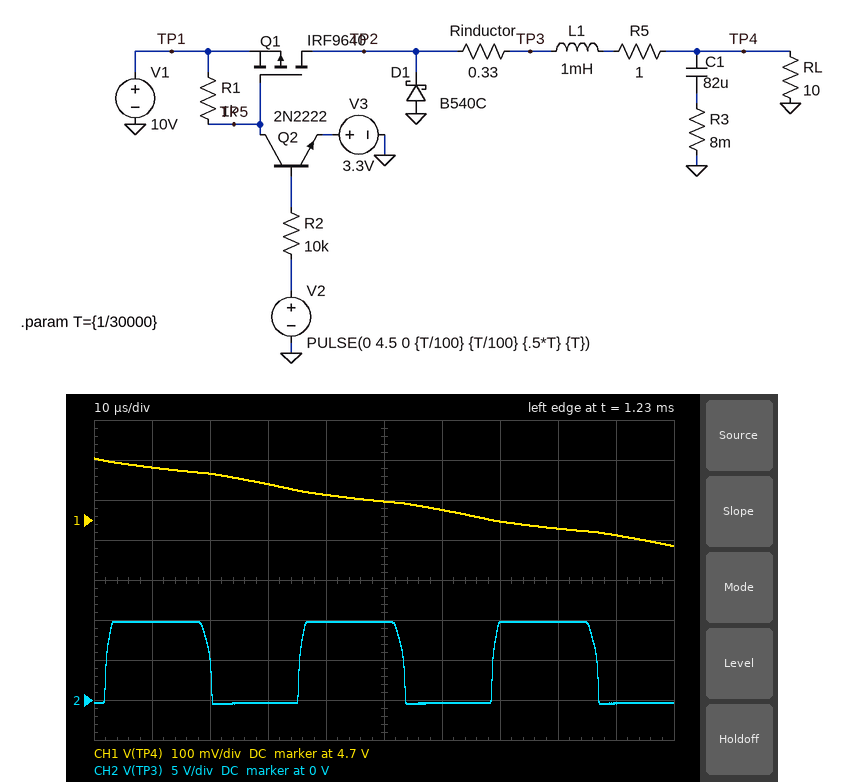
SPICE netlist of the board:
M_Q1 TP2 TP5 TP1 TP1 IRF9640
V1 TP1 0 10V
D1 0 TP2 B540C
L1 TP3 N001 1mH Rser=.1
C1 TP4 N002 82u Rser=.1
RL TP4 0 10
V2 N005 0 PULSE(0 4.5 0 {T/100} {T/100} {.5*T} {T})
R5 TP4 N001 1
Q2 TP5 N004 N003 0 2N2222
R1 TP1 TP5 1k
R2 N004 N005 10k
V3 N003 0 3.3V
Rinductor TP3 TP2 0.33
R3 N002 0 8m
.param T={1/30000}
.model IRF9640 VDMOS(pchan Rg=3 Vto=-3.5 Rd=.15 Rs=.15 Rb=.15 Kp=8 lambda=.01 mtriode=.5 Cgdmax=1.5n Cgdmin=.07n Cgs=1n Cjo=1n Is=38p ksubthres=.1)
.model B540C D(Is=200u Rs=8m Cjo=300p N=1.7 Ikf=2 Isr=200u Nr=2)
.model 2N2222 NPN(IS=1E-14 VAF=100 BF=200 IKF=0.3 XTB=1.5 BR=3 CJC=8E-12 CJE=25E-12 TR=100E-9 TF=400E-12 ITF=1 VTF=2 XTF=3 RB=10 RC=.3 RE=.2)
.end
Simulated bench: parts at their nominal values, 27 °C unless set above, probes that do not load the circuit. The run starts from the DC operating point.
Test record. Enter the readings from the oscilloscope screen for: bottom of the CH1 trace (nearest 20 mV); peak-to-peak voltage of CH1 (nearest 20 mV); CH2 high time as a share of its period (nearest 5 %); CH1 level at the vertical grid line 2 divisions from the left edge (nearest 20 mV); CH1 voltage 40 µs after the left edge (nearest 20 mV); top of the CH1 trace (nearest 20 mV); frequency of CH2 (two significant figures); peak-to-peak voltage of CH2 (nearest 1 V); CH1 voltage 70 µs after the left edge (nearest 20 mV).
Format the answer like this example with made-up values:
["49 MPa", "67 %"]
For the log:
["4.64 V", "220 mV", "55 %", "4.82 V", "4.76 V", "4.86 V", "30 kHz", "10 V", "4.70 V"]
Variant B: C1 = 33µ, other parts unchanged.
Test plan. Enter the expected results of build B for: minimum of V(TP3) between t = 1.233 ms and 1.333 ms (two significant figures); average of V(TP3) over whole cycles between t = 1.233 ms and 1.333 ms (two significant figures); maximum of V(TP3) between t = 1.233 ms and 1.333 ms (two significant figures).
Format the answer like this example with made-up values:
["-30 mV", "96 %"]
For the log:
["-520 mV", "4.8 V", "9.7 V"]
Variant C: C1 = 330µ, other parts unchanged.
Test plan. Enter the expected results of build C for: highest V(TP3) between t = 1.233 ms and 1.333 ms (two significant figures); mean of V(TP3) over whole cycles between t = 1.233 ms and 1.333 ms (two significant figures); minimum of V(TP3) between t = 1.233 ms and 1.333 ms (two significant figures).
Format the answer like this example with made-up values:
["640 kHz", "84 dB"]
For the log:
["9.2 V", "4.3 V", "-820 mV"]
